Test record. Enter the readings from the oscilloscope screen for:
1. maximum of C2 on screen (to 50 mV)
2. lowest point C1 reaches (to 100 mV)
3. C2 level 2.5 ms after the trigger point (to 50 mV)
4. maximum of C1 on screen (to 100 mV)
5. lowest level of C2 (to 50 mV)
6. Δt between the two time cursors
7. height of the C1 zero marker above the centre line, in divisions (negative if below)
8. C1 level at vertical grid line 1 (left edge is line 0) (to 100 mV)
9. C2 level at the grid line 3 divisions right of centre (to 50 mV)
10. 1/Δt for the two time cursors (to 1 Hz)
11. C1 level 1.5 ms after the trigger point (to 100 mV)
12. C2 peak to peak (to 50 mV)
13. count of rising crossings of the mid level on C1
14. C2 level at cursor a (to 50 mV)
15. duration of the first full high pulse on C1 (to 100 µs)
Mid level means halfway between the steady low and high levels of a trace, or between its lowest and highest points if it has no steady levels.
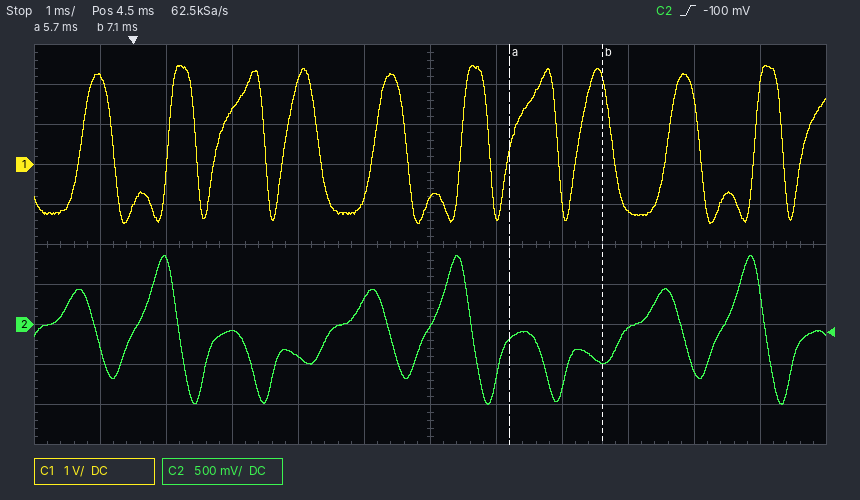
850 mV
-1.5 V
-400 mV
2.5 V
-1.00 V
1.4 ms
+2.0 div
2.2 V
-50 mV
714 Hz
1.4 V
1.85 V
11
-200 mV
500 µs
